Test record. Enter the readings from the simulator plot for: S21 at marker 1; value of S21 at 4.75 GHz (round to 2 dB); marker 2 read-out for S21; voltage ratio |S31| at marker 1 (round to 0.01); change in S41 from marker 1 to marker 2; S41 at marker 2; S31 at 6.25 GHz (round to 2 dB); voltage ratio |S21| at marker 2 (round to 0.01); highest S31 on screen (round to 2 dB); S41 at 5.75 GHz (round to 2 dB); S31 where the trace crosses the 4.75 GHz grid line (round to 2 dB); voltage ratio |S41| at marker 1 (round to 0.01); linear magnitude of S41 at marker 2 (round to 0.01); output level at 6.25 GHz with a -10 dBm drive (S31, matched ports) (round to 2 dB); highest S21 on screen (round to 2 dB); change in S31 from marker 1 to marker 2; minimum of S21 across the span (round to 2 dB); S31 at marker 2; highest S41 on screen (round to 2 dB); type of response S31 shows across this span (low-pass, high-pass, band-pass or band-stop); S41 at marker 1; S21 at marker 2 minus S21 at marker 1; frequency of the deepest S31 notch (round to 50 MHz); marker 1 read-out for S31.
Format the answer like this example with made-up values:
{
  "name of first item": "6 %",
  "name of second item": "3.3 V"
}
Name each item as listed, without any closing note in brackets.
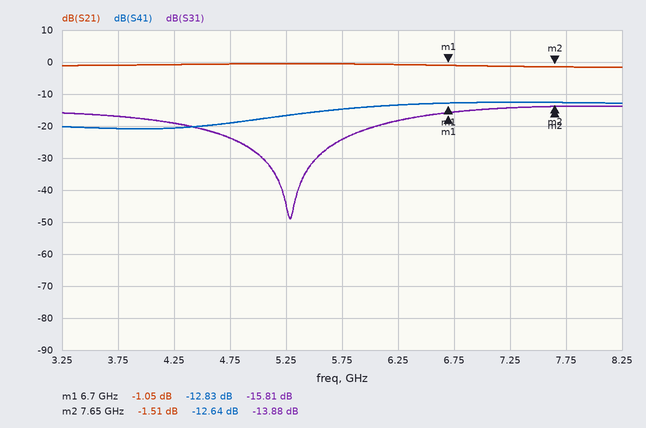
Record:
{
  "S21 at marker 1": "-1.05 dB",
  "value of S21 at 4.75 GHz": "0 dB",
  "marker 2 read-out for S21": "-1.51 dB",
  "voltage ratio |S31| at marker 1": "0.16",
  "change in S41 from marker 1 to marker 2": "0.19 dB",
  "S41 at marker 2": "-12.64 dB",
  "S31 at 6.25 GHz": "-18 dB",
  "voltage ratio |S21| at marker 2": "0.84",
  "highest S31 on screen": "-14 dB",
  "S41 at 5.75 GHz": "-14 dB",
  "S31 where the trace crosses the 4.75 GHz grid line": "-24 dB",
  "voltage ratio |S41| at marker 1": "0.23",
  "linear magnitude of S41 at marker 2": "0.23",
  "output level at 6.25 GHz with a -10 dBm drive (S31, matched ports)": "-28 dBm",
  "highest S21 on screen": "0 dB",
  "change in S31 from marker 1 to marker 2": "1.93 dB",
  "minimum of S21 across the span": "-2 dB",
  "S31 at marker 2": "-13.88 dB",
  "highest S41 on screen": "-12 dB",
  "type of response S31 shows across this span": "band-stop",
  "S41 at marker 1": "-12.83 dB",
  "S21 at marker 2 minus S21 at marker 1": "-0.46 dB",
  "frequency of the deepest S31 notch": "5.30 GHz",
  "marker 1 read-out for S31": "-15.81 dB"
}
